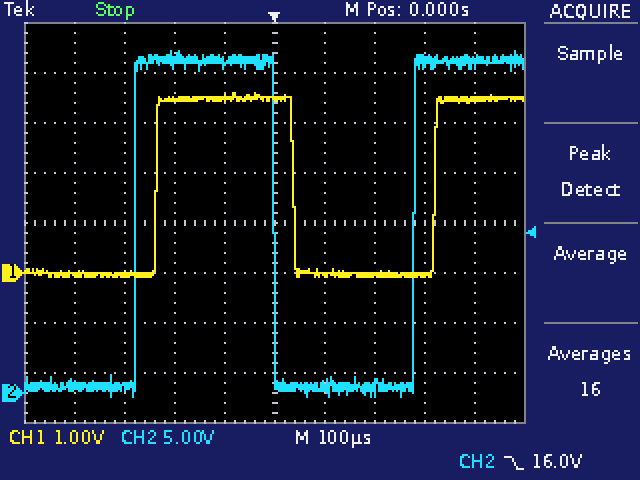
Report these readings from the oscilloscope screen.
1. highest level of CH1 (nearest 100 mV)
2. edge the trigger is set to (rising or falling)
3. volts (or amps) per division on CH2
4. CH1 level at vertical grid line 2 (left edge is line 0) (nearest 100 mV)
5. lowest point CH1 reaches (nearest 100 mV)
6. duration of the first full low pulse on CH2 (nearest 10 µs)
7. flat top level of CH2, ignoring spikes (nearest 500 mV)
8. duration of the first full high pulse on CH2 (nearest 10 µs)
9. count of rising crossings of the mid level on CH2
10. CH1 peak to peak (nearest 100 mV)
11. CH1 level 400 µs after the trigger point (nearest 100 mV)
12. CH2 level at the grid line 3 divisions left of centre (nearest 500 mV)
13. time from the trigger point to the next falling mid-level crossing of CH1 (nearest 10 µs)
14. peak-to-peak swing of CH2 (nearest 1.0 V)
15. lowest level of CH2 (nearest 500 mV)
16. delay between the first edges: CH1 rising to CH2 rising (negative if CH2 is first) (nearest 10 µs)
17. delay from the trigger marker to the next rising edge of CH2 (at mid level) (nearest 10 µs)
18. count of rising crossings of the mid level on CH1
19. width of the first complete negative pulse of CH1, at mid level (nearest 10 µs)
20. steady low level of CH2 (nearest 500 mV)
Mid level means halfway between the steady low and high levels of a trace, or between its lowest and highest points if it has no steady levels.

3.6 V
falling
5 V
0.0 V
-100 mV
280 µs
33.5 V
280 µs
2
3.7 V
3.5 V
500 mV
40 µs
35.0 V
-500 mV
-40 µs
280 µs
2
280 µs
500 mV
